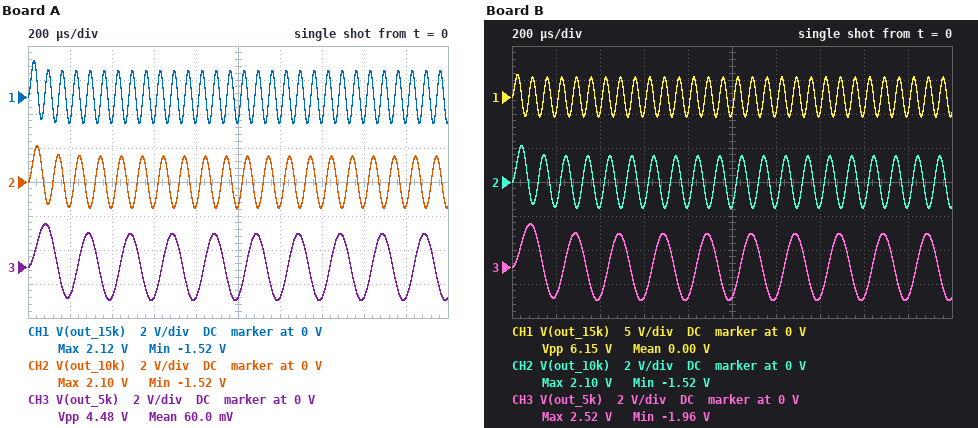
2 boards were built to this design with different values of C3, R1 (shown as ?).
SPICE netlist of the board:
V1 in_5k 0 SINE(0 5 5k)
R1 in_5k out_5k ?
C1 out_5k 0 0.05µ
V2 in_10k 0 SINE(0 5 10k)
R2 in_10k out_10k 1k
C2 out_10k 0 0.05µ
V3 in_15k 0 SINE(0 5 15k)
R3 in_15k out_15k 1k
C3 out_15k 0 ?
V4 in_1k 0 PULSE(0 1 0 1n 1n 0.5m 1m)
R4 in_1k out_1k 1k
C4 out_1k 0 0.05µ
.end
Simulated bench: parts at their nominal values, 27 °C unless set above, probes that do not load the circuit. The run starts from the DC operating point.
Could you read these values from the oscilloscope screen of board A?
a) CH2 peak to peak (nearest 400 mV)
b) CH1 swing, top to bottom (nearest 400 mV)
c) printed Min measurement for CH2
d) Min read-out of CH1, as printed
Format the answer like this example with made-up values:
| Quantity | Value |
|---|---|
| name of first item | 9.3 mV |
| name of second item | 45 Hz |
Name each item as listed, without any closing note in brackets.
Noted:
| Quantity | Value |
|---|---|
| CH2 peak to peak | 3.6 V |
| CH1 swing, top to bottom | 3.6 V |
| printed Min measurement for CH2 | -1.52 V |
| Min read-out of CH1, as printed | -1.52 V |
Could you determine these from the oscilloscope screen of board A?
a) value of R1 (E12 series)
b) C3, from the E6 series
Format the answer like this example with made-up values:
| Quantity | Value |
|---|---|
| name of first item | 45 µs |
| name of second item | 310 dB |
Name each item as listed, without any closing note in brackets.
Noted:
| Quantity | Value |
|---|---|
| value of R1 | 1.5 kΩ |
| C3, from the E6 series | 33 nF |
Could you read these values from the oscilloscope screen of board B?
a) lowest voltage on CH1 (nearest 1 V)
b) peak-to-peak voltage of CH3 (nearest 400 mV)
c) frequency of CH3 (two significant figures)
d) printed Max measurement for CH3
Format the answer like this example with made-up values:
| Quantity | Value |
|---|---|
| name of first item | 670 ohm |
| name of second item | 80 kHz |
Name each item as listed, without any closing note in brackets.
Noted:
| Quantity | Value |
|---|---|
| lowest voltage on CH1 | -3 V |
| peak-to-peak voltage of CH3 | 4.4 V |
| frequency of CH3 | 5.0 kHz |
| printed Max measurement for CH3 | 2.52 V |
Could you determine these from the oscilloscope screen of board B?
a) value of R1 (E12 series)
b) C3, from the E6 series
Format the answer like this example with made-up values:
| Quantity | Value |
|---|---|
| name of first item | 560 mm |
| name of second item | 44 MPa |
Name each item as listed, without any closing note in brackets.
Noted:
| Quantity | Value |
|---|---|
| value of R1 | 1.5 kΩ |
| C3, from the E6 series | 15 nF |
